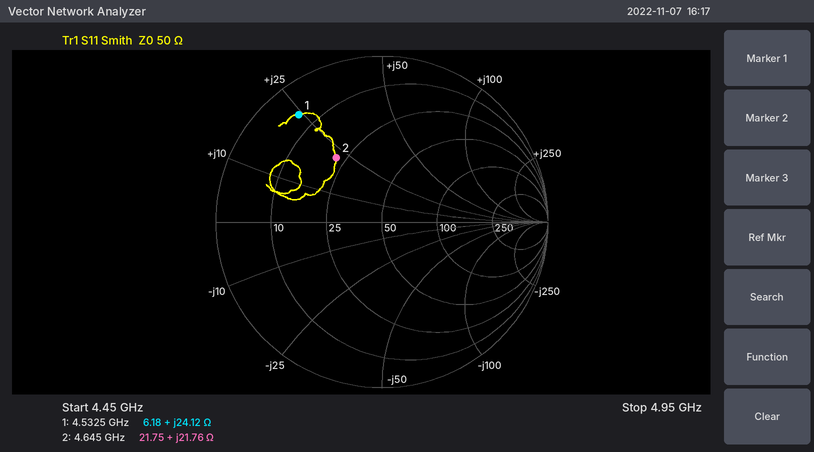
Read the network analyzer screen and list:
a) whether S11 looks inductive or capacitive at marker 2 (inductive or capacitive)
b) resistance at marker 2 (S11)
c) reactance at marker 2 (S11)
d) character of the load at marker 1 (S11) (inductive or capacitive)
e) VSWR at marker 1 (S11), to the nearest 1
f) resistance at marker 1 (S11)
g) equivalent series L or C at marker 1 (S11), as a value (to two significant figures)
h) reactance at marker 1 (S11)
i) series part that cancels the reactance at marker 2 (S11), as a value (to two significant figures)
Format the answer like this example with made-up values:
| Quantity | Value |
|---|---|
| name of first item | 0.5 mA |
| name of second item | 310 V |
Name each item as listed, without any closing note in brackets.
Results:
| Quantity | Value |
|---|---|
| whether S11 looks inductive or capacitive at marker 2 | inductive |
| resistance at marker 2 | 21.75 Ω |
| reactance at marker 2 | +21.76 Ω |
| character of the load at marker 1 (S11) | inductive |
| VSWR at marker 1 (S11), to the nearest 1 | 10 |
| resistance at marker 1 | 6.18 Ω |
| equivalent series L or C at marker 1 (S11), as a value | 850 pH |
| reactance at marker 1 | +24.12 Ω |
| series part that cancels the reactance at marker 2 (S11), as a value | 1.6 pF |
